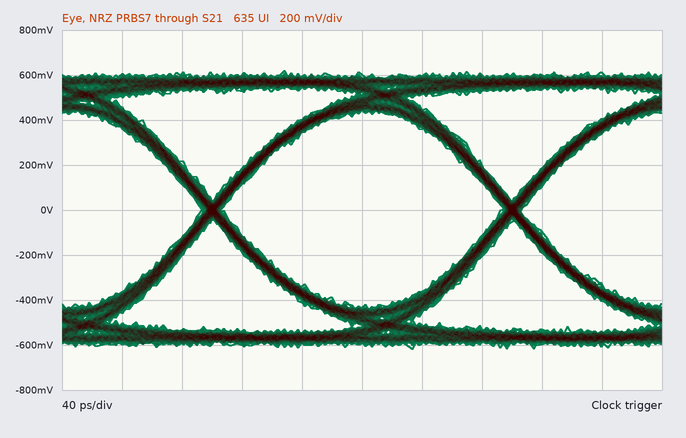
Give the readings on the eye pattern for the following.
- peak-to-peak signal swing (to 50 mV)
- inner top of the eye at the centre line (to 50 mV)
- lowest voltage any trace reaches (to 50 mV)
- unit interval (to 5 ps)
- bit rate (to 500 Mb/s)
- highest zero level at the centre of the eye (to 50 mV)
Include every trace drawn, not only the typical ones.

1.25 V
450 mV
-600 mV
200 ps
5.0 Gb/s
-450 mV
